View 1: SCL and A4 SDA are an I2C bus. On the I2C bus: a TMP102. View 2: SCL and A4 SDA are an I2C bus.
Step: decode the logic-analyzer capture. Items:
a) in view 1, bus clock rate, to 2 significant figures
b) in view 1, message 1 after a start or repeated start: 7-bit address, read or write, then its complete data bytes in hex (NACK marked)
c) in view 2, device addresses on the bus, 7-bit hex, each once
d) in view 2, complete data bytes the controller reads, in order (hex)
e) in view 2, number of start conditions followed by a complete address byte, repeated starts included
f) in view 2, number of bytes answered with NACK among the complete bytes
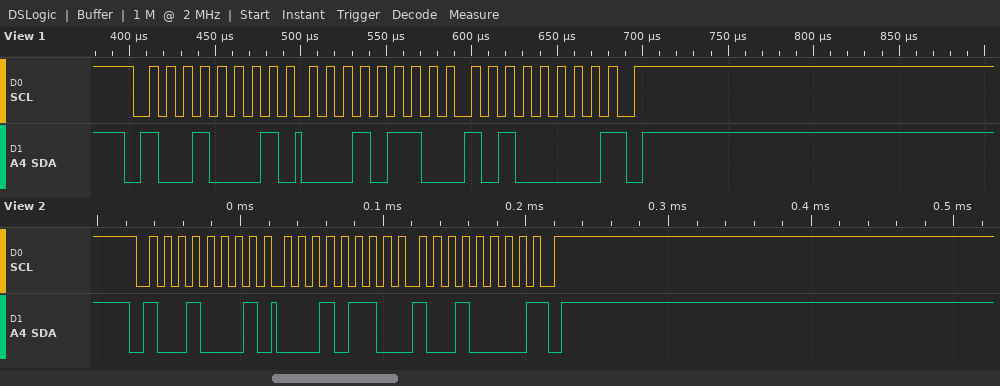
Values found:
100 kHz
0x48 read: 16 A0 NACK
0x48
16 90
1
1
